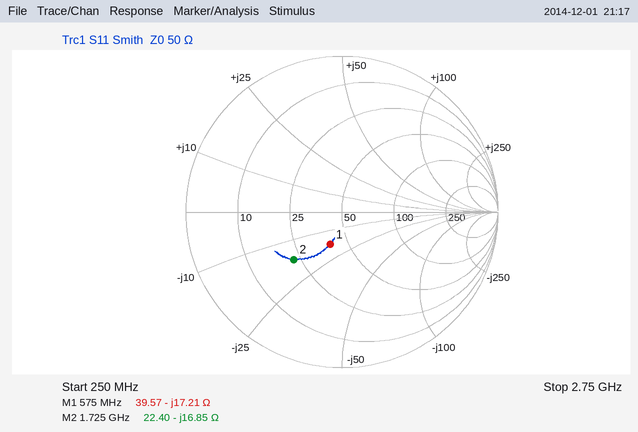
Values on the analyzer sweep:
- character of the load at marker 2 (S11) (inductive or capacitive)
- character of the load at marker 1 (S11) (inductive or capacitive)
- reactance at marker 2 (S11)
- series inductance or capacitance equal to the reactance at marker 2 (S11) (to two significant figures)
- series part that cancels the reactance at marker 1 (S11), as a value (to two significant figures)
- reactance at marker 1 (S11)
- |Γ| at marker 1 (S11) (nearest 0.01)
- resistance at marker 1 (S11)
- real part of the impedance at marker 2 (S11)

capacitive
capacitive
-16.85 Ω
5.5 pF
4.8 nH
-17.21 Ω
0.22
39.57 Ω
22.40 Ω
